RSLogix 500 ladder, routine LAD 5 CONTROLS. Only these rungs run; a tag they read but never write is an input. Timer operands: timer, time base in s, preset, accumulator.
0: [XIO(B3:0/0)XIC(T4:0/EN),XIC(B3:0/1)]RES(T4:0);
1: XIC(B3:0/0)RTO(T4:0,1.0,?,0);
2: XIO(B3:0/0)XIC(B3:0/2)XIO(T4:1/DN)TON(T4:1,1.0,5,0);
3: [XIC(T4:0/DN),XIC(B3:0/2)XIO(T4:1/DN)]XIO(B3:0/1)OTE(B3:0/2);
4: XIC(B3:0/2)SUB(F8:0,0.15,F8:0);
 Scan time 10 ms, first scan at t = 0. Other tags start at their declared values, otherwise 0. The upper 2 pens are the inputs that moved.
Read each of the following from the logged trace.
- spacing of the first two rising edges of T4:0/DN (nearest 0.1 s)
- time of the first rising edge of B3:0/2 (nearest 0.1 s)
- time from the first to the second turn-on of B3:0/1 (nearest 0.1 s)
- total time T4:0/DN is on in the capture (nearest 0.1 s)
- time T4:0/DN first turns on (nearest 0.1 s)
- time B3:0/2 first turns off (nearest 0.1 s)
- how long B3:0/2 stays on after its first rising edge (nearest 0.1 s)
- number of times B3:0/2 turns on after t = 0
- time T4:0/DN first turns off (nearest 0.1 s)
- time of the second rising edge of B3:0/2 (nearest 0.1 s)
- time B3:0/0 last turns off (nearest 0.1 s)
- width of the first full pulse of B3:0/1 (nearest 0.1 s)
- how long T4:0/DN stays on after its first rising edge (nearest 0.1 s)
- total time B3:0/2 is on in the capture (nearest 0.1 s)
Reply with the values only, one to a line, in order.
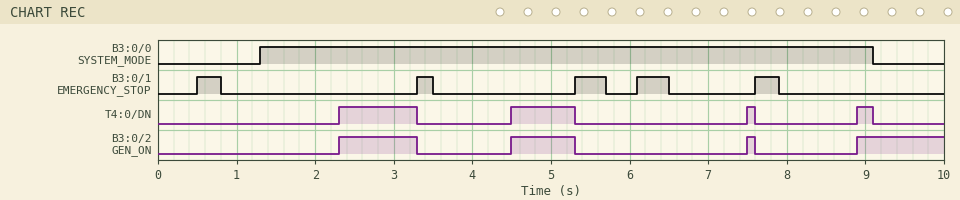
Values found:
2.2 s
2.3 s
2.8 s
2.1 s
2.3 s
3.3 s
1.0 s
4
3.3 s
4.5 s
9.1 s
0.3 s
1.0 s
3.0 s
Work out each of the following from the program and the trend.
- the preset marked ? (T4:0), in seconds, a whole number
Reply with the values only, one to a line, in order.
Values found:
1 s
